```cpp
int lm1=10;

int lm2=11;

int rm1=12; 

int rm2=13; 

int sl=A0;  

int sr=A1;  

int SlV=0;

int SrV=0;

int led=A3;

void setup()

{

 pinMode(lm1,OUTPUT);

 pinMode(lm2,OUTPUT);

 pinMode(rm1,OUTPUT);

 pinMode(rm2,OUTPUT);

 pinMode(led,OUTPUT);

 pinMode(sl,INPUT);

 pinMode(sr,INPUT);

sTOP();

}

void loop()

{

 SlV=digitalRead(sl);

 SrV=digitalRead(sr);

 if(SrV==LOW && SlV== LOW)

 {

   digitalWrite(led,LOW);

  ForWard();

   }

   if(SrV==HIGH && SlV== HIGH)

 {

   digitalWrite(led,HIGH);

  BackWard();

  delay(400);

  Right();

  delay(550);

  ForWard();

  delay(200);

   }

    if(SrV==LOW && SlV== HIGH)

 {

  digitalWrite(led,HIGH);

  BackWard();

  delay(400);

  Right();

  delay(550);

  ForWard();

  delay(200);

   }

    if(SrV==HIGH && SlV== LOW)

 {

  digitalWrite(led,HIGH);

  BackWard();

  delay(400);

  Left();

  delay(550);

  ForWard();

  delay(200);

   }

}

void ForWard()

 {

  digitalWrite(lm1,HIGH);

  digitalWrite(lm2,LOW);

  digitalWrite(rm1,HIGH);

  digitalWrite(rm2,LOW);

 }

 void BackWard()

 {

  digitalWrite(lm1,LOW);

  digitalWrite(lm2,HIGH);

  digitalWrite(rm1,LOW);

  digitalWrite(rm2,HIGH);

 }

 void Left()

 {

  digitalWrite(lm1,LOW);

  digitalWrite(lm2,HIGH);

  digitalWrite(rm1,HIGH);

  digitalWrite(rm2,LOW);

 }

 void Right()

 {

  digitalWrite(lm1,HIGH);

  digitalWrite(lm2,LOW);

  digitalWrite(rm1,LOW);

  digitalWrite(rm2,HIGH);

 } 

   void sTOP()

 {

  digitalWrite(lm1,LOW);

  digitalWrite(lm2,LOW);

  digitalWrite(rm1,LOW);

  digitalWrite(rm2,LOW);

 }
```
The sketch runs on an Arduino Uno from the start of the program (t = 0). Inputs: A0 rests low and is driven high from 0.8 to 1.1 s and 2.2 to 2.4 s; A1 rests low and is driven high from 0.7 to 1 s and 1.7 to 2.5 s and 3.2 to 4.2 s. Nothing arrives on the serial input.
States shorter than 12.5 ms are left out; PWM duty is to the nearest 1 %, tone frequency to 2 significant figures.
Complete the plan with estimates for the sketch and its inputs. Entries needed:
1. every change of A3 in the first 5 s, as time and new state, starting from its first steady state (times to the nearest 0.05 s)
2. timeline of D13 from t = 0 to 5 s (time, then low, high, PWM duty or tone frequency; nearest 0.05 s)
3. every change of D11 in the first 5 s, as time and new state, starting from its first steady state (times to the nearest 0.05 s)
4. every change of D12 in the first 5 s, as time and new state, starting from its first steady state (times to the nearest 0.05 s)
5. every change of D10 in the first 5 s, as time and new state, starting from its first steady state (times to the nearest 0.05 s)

0 s low; 0.7 s high; 3 s low; 3.2 s high; 4.35 s low
0 s low; 0.7 s high; 1.1 s low; 1.85 s high; 2.25 s low; 3.2 s high; 3.6 s low
0 s low; 0.7 s high; 1.65 s low; 1.85 s high; 2.8 s low; 3.2 s high; 4.15 s low
0 s high; 0.7 s low; 1.1 s high; 1.85 s low; 2.25 s high; 3.2 s low; 3.6 s high
0 s high; 0.7 s low; 1.65 s high; 1.85 s low; 2.8 s high; 3.2 s low; 4.15 s high
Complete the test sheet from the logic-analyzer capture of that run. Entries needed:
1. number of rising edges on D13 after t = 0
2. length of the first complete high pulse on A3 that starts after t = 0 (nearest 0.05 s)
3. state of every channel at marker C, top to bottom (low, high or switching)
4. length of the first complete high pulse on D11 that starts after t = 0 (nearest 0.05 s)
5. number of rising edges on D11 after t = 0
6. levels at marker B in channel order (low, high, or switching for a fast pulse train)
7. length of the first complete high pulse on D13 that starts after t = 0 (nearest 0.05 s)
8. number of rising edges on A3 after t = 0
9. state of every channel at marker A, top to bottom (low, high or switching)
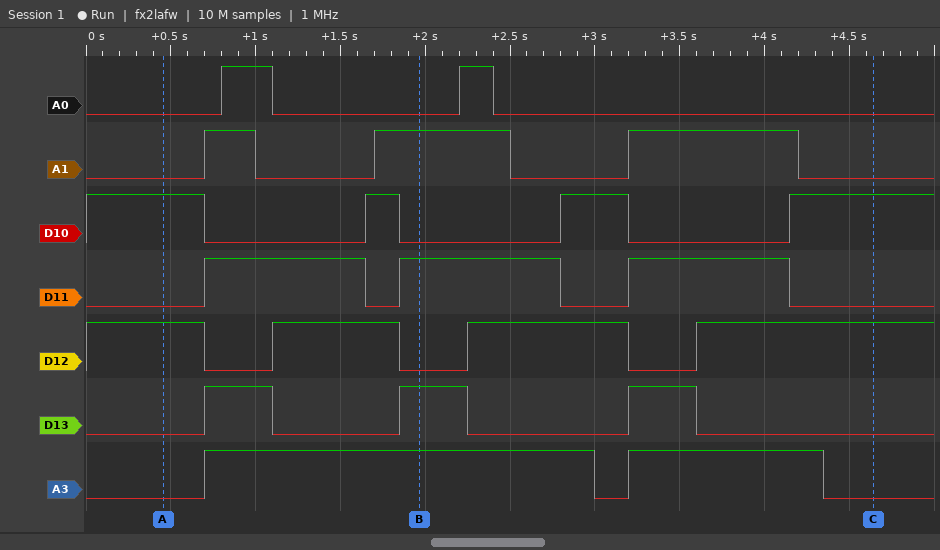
3
2.30 s
A0 low, A1 low, D10 high, D11 low, D12 high, D13 low, A3 low
0.95 s
3
A0 low, A1 high, D10 low, D11 high, D12 low, D13 high, A3 high
0.40 s
2
A0 low, A1 low, D10 high, D11 low, D12 high, D13 low, A3 low
